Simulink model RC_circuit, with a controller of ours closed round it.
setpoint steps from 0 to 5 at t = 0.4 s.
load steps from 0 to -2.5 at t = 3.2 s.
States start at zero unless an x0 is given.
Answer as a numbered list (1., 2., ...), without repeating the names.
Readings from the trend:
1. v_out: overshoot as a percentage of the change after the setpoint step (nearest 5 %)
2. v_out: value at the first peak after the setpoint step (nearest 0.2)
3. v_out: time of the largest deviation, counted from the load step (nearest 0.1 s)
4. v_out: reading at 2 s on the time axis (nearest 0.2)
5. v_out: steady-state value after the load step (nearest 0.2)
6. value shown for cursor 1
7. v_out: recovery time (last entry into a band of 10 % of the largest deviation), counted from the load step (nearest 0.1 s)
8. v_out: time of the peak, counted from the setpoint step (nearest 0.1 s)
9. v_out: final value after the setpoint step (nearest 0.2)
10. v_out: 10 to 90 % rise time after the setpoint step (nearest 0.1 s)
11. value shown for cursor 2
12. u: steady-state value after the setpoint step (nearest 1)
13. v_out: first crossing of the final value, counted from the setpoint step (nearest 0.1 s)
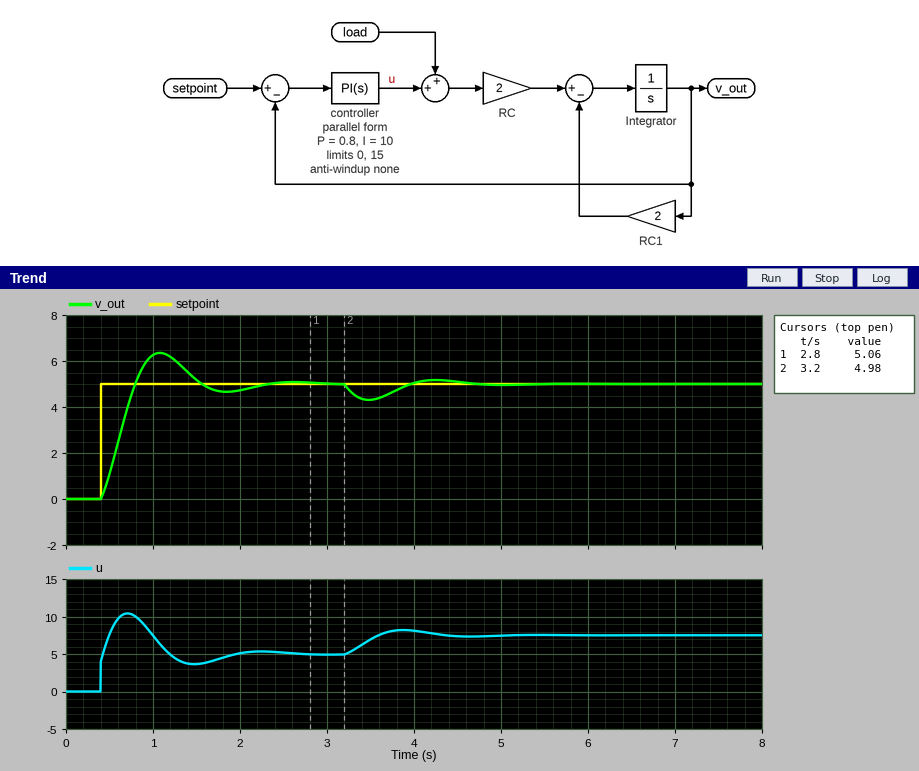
1. 25 %
2. 6.4
3. 0.3 s
4. 4.8
5. 5.0
6. 5.06
7. 1.4 s
8. 0.7 s
9. 5.0
10. 0.3 s
11. 4.98
12. 5
13. 0.4 s
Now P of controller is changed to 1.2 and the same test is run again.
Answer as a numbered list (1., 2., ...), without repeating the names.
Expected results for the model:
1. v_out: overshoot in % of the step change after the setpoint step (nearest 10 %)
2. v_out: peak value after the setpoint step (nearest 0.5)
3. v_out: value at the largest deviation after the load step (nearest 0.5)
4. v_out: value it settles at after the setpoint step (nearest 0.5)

1. 20 %
2. 6.0
3. 4.5
4. 5.0
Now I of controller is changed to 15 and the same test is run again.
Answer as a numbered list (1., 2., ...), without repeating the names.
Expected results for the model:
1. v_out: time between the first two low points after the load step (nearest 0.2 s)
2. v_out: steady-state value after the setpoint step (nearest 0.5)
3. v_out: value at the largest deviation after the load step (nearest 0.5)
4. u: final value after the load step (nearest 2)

1. 1.2 s
2. 5.0
3. 4.5
4. 8
